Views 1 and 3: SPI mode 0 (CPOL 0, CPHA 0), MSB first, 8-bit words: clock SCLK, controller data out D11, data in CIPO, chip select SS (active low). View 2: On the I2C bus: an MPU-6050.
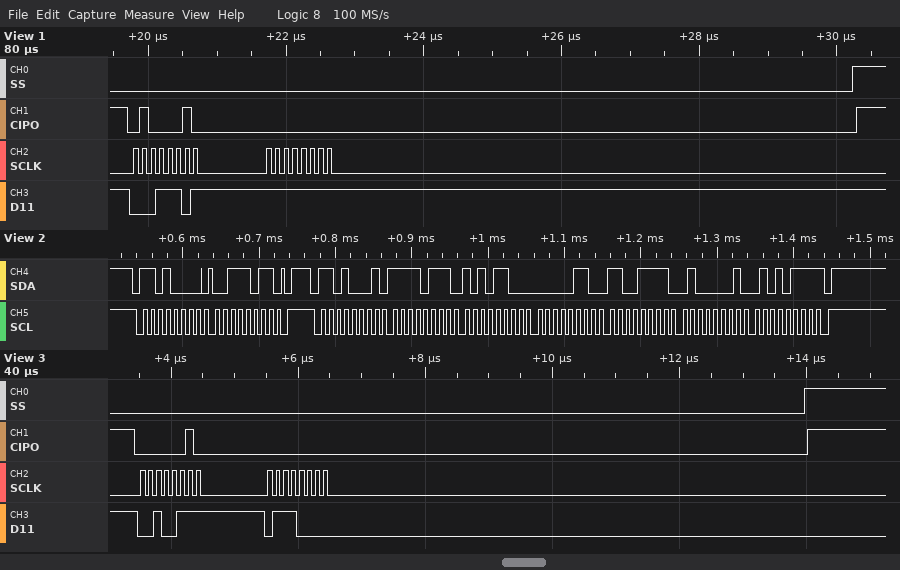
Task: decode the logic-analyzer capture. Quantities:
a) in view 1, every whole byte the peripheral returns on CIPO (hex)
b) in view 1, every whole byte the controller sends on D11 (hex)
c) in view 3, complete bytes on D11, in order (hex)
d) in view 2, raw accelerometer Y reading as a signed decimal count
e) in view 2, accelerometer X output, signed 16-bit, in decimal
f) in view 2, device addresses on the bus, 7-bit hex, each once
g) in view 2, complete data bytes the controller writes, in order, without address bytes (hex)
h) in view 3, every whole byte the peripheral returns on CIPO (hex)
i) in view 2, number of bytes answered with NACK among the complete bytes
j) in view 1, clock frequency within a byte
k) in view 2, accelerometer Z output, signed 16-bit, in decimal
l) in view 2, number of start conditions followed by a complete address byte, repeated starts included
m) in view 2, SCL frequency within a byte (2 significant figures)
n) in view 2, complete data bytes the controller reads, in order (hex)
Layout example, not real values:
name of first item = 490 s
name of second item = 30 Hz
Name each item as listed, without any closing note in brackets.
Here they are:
in view 1, every whole byte the peripheral returns on CIPO = 0x42 0x00
in view 1, every whole byte the controller sends on D11 = 0x1D 0xFF
in view 3, complete bytes on D11, in order = 0x27 0x70
in view 2, raw accelerometer Y reading as a signed decimal count = 1743
in view 2, accelerometer X output, signed 16-bit, in decimal = -2132
in view 2, device addresses on the bus, 7-bit hex, each once = 0x68
in view 2, complete data bytes the controller writes, in order, without address bytes = 3B
in view 3, every whole byte the peripheral returns on CIPO = 0x02 0x00
in view 2, number of bytes answered with NACK among the complete bytes = 1
in view 1, clock frequency within a byte = 8 MHz
in view 2, accelerometer Z output, signed 16-bit, in decimal = 16727
in view 2, number of start conditions followed by a complete address byte, repeated starts included = 2
in view 2, SCL frequency within a byte = 100 kHz
in view 2, complete data bytes the controller reads, in order = F7 AC 06 CF 41 57
